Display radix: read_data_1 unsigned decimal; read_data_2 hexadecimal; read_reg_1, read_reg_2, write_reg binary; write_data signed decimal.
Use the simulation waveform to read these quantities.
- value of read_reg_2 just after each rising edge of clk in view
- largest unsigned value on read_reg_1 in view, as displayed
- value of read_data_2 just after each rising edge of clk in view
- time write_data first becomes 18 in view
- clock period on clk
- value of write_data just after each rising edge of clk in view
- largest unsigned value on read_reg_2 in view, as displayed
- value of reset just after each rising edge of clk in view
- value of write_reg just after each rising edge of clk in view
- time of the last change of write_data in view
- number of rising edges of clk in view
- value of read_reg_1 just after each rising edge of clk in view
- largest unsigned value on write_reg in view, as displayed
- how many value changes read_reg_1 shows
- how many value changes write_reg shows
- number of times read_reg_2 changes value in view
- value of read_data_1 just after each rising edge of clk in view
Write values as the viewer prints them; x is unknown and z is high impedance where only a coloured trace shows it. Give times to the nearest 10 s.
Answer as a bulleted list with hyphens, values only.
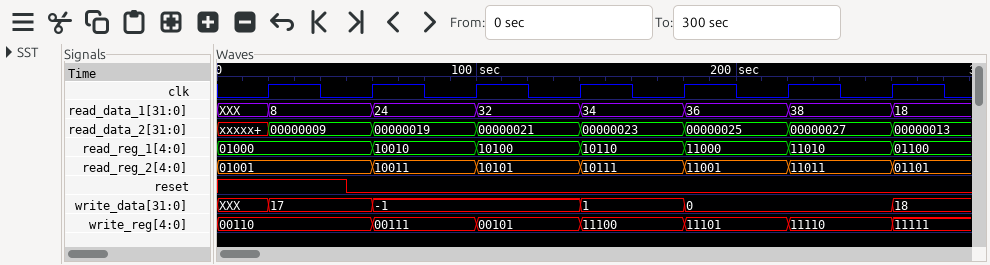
- 01001, 10011, 10101, 10111, 11001, 11011, 01101
- 11010
- 00000009, 00000019, 00000021, 00000023, 00000025, 00000027, 00000013
- 260 s
- 40 s
- 17, -1, -1, 1, 0, 0, 18
- 11011
- 1 0 0 0 0 0 0
- 00110, 00111, 00101, 11100, 11101, 11110, 11111
- 260 s
- 7
- 01000, 10010, 10100, 10110, 11000, 11010, 01100
- 11111
- 6
- 6
- 6
- 8, 24, 32, 34, 36, 38, 18
